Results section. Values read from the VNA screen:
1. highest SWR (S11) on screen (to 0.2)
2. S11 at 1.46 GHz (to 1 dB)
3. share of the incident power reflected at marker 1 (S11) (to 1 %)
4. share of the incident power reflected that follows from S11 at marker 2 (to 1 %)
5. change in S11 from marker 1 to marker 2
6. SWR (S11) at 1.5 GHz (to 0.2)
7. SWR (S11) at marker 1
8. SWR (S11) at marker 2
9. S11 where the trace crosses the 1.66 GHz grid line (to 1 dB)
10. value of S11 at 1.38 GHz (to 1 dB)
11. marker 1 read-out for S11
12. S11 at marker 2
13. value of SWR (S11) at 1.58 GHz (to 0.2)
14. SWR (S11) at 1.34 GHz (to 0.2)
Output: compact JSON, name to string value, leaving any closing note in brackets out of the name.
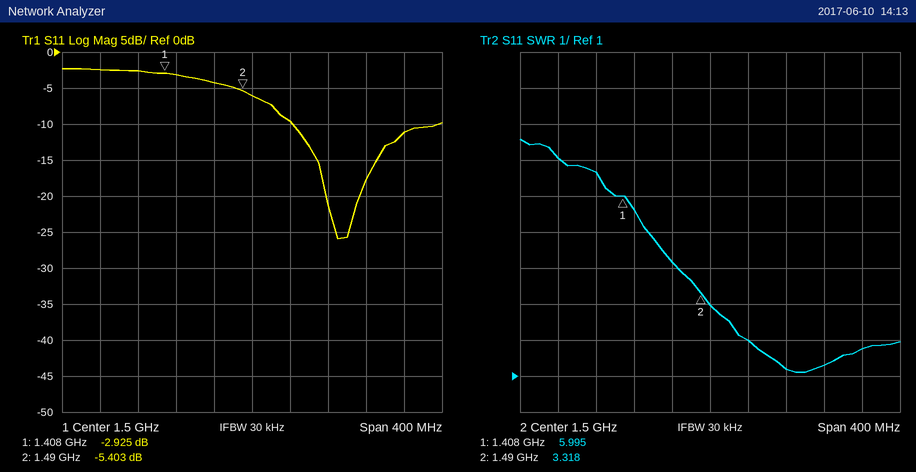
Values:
{"highest SWR (S11) on screen": "7.6", "S11 at 1.46 GHz": "-4 dB", "share of the incident power reflected at marker 1 (S11)": "51 %", "share of the incident power reflected that follows from S11 at marker 2": "29 %", "change in S11 from marker 1 to marker 2": "-2.478 dB", "SWR (S11) at 1.5 GHz": "3.0", "SWR (S11) at marker 1": "5.995", "SWR (S11) at marker 2": "3.318", "S11 where the trace crosses the 1.66 GHz grid line": "-11 dB", "value of S11 at 1.38 GHz": "-3 dB", "marker 1 read-out for S11": "-2.925 dB", "S11 at marker 2": "-5.403 dB", "value of SWR (S11) at 1.58 GHz": "1.2", "SWR (S11) at 1.34 GHz": "7.0"}
